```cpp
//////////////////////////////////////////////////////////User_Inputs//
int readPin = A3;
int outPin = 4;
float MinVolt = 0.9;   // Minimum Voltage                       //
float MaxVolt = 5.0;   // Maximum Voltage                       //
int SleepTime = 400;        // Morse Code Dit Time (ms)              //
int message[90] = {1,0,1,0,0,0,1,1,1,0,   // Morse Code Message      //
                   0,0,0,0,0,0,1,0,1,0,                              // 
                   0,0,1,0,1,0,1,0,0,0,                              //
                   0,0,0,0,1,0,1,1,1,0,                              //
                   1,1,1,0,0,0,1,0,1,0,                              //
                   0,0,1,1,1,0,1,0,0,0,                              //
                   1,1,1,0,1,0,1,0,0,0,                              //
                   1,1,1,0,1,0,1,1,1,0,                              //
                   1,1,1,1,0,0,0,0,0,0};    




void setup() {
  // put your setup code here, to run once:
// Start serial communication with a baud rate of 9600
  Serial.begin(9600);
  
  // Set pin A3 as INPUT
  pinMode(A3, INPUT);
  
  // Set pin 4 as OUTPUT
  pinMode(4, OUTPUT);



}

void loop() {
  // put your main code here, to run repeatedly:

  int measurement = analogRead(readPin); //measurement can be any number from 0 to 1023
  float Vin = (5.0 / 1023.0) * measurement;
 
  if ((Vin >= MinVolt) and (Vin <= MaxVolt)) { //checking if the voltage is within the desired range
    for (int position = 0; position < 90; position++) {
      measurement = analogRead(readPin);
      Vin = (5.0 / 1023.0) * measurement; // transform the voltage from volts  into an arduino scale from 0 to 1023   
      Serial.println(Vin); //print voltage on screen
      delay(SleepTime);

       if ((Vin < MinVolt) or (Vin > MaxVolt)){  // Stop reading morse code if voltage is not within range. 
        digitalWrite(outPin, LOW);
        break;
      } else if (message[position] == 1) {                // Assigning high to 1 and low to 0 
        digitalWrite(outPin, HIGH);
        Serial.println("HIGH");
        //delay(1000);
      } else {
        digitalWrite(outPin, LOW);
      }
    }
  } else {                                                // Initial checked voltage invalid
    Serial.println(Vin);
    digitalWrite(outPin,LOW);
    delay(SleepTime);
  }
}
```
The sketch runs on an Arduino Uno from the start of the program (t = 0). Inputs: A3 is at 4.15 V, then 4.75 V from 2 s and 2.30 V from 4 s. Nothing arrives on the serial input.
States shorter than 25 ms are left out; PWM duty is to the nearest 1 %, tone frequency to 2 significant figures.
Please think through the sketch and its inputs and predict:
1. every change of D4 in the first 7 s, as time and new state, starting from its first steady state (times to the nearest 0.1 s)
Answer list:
0 s low; 0.4 s high; 0.8 s low; 1.2 s high; 1.6 s low; 2.8 s high; 4 s low; 6.8 s high
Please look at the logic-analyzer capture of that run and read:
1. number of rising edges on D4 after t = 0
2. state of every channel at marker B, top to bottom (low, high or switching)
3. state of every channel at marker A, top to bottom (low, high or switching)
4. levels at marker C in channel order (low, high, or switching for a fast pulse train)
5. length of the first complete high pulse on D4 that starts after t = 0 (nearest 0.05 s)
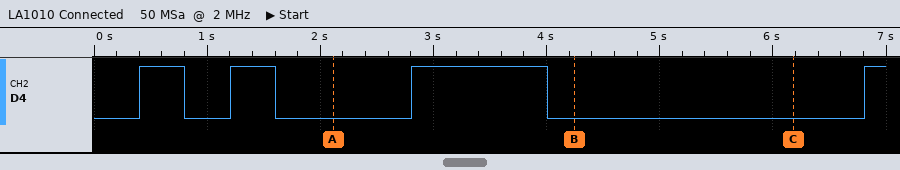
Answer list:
4
D4 low
D4 low
D4 low
0.40 s
